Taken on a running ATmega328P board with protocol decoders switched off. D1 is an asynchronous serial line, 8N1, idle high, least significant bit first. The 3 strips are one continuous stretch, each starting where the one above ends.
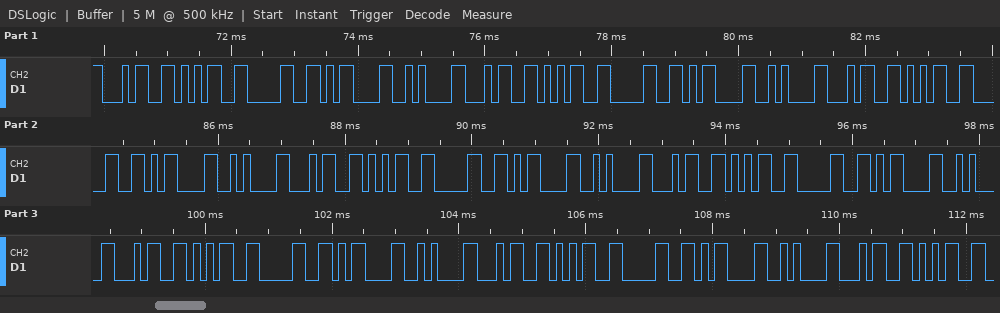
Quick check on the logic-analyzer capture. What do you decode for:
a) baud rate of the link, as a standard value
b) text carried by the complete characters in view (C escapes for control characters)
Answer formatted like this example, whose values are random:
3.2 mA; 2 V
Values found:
9600 baud; "450\r\n450\r\n450\r\n450\r\n450\r\n450\r\n450\r\n45"
